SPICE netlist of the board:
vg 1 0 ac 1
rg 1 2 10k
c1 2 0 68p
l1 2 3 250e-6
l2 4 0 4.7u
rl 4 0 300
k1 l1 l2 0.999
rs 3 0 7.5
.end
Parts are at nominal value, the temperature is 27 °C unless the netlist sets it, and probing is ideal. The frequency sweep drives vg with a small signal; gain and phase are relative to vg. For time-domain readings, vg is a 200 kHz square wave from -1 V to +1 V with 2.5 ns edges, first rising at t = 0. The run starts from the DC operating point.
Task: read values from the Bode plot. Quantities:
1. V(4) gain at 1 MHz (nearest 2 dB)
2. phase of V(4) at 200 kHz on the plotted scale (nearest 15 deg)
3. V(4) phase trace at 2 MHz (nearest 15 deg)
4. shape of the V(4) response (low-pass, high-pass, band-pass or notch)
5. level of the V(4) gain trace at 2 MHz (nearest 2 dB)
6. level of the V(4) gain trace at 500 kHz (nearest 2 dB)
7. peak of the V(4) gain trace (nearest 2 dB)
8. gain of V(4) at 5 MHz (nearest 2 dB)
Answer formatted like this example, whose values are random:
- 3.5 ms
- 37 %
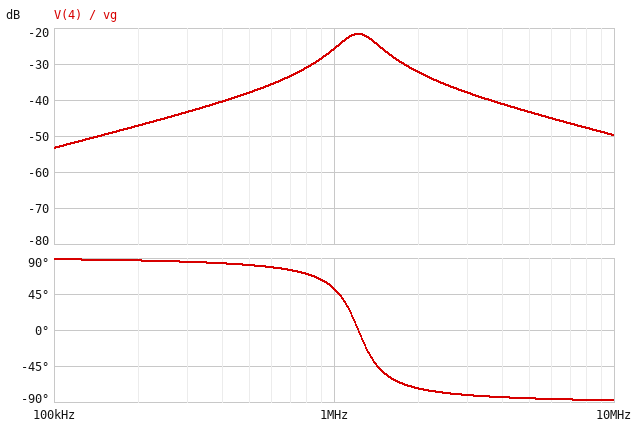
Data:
- -26 dB
- 90 deg
- -75 deg
- band-pass
- -32 dB
- -38 dB
- -22 dB
- -44 dB
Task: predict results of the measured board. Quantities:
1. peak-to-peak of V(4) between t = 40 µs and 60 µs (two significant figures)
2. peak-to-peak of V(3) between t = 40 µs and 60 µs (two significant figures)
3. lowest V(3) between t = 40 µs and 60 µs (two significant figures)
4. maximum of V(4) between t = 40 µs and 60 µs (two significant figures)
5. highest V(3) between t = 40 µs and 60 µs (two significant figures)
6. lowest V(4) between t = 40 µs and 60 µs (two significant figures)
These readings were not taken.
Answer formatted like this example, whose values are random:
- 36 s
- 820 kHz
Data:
- 80 mV
- 3.2 mV
- -1.6 mV
- 40 mV
- 1.6 mV
- -40 mV
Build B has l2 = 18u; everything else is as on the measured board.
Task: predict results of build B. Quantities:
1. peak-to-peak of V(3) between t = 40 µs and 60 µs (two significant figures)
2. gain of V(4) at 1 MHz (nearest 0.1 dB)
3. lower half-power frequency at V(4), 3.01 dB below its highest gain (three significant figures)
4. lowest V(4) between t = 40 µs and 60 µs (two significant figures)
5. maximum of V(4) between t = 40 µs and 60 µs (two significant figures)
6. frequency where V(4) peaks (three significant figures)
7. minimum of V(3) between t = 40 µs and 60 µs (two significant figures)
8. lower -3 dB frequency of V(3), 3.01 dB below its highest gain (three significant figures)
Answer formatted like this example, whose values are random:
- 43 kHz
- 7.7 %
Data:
- 2.6 mV
- -23.5 dB
- 885 kHz
- -67 mV
- 67 mV
- 1.22 MHz
- -1.3 mV
- 591 kHz
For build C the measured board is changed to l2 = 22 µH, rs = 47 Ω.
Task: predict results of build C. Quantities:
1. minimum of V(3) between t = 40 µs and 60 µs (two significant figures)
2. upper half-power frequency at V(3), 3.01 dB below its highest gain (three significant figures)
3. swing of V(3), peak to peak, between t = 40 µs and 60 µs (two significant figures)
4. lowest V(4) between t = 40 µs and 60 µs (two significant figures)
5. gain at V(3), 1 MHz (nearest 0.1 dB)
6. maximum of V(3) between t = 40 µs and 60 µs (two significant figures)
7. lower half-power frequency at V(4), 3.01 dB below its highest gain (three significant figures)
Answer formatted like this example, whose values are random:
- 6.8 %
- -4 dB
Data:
- -7.7 mV
- 1.51 MHz
- 15 mV
- -69 mV
- -42.8 dB
- 7.7 mV
- 833 kHz
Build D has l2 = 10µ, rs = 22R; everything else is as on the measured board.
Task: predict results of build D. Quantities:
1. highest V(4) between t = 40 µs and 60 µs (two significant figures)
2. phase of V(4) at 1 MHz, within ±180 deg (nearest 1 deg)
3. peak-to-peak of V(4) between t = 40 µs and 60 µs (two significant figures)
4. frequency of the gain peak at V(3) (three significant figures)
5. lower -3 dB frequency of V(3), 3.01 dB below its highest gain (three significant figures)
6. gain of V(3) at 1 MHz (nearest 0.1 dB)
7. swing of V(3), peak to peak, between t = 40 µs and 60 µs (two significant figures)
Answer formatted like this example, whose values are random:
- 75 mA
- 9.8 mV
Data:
- 55 mV
- 41 deg
- 110 mV
- 1.16 MHz
- 829 kHz
- -46.9 dB
- 8.7 mV
